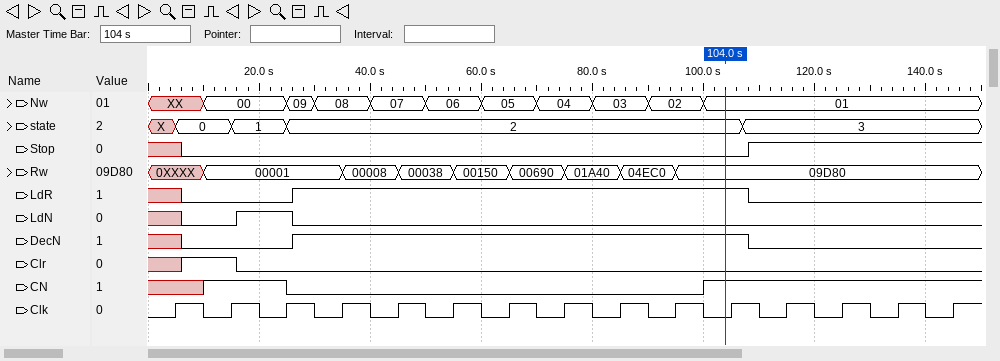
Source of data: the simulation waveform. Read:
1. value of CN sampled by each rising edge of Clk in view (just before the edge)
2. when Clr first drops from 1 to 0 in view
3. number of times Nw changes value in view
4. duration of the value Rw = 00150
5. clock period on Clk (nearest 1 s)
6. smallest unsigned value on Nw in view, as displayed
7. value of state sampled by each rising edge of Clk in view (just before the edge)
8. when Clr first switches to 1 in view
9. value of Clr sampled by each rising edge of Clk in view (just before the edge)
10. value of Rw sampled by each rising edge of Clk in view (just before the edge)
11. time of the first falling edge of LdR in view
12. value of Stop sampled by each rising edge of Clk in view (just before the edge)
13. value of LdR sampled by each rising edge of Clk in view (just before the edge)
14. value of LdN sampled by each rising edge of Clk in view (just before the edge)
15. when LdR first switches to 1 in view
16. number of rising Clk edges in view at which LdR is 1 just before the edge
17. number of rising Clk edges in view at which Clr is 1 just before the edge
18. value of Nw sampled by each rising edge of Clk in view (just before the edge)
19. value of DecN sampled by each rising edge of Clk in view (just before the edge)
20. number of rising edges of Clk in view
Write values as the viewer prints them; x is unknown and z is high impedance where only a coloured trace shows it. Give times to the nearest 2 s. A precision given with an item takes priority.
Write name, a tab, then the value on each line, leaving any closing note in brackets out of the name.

value of CN sampled by each rising edge of Clk in view	x 1 1 0 0 0 0 0 0 0 1 1 1 1 1
when Clr first drops from 1 to 0 in view	16 s
number of times Nw changes value in view	10
duration of the value Rw = 00150	10 s
clock period on Clk	10 s
smallest unsigned value on Nw in view, as displayed	00
value of state sampled by each rising edge of Clk in view	X, 0, 1, 2, 2, 2, 2, 2, 2, 2, 2, 3, 3, 3, 3
when Clr first switches to 1 in view	6 s
value of Clr sampled by each rising edge of Clk in view	x 1 0 0 0 0 0 0 0 0 0 0 0 0 0
value of Rw sampled by each rising edge of Clk in view	0XXXX, 00001, 00001, 00001, 00008, 00038, 00150, 00690, 01A40, 04EC0, 09D80, 09D80, 09D80, 09D80, 09D80
time of the first falling edge of LdR in view	108 s
value of Stop sampled by each rising edge of Clk in view	x 0 0 0 0 0 0 0 0 0 0 1 1 1 1
value of LdR sampled by each rising edge of Clk in view	x 0 0 1 1 1 1 1 1 1 1 0 0 0 0
value of LdN sampled by each rising edge of Clk in view	x 0 1 0 0 0 0 0 0 0 0 0 0 0 0
when LdR first switches to 1 in view	26 s
number of rising Clk edges in view at which LdR is 1 just before the edge	8
number of rising Clk edges in view at which Clr is 1 just before the edge	1
value of Nw sampled by each rising edge of Clk in view	XX, 00, 00, 08, 07, 06, 05, 04, 03, 02, 01, 01, 01, 01, 01
value of DecN sampled by each rising edge of Clk in view	x 0 0 1 1 1 1 1 1 1 1 0 0 0 0
number of rising edges of Clk in view	15
